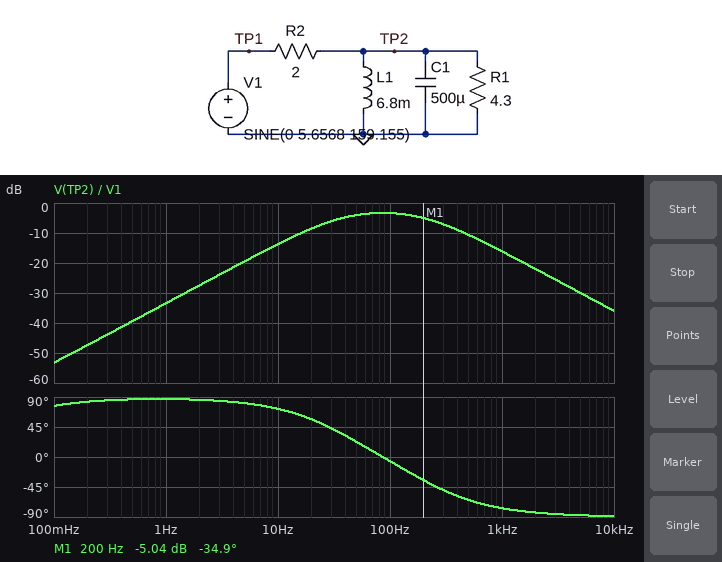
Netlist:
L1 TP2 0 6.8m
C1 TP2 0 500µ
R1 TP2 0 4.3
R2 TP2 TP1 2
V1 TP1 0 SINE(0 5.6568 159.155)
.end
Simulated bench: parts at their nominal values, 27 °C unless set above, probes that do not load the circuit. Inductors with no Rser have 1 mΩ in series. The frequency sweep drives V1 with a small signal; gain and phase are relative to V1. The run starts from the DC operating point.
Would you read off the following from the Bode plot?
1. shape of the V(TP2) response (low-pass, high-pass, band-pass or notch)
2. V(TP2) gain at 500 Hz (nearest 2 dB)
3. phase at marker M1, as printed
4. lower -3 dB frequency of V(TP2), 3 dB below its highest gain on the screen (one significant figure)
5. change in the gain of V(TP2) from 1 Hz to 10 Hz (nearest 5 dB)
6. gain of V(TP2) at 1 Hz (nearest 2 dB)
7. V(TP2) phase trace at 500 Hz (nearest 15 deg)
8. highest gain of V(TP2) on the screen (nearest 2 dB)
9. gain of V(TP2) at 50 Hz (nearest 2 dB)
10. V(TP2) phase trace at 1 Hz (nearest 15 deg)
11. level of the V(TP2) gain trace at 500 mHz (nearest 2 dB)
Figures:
band-pass
-10 dB
-34.9 deg
30 Hz
20 dB
-34 dB
-60 deg
-4 dB
-4 dB
90 deg
-40 dB
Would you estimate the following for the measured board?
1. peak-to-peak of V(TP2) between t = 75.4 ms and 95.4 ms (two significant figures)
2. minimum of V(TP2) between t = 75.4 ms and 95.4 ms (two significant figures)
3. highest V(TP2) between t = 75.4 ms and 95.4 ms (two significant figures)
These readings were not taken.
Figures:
7.0 V
-3.5 V
3.5 V
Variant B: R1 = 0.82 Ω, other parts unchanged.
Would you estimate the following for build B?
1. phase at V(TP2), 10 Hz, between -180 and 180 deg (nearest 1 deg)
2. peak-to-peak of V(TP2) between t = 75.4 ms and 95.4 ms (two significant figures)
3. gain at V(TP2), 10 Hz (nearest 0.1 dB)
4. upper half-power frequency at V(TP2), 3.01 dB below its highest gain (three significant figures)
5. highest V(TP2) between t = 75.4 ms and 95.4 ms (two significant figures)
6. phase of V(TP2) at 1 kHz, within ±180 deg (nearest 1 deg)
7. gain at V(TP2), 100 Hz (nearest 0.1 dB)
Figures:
53 deg
3.2 V
-15.2 dB
561 Hz
1.6 V
-61 deg
-10.7 dB
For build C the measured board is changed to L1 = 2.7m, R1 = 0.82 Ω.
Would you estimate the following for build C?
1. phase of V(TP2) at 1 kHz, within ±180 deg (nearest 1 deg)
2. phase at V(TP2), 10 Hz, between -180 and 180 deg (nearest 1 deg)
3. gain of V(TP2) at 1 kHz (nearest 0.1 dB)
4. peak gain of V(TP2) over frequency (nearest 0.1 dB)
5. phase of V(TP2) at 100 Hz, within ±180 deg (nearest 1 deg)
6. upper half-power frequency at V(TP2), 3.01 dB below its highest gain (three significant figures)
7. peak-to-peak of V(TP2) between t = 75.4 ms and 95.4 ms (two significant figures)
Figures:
-61 deg
73 deg
-17.0 dB
-10.7 dB
9 deg
580 Hz
3.3 V
